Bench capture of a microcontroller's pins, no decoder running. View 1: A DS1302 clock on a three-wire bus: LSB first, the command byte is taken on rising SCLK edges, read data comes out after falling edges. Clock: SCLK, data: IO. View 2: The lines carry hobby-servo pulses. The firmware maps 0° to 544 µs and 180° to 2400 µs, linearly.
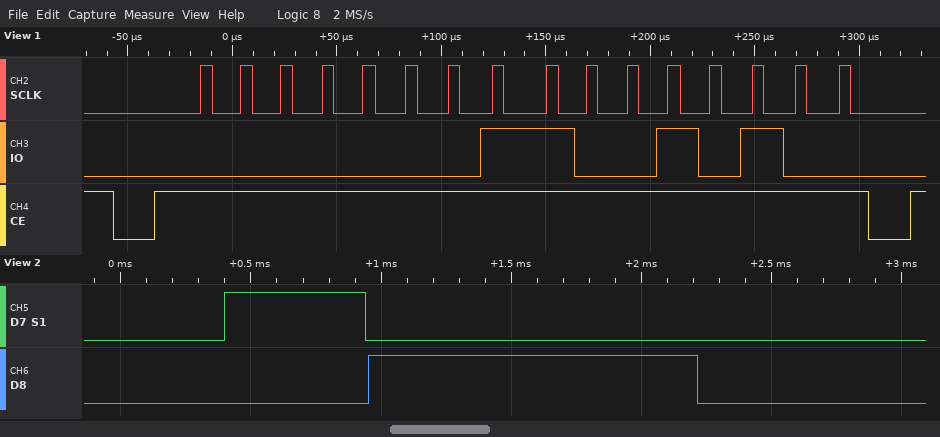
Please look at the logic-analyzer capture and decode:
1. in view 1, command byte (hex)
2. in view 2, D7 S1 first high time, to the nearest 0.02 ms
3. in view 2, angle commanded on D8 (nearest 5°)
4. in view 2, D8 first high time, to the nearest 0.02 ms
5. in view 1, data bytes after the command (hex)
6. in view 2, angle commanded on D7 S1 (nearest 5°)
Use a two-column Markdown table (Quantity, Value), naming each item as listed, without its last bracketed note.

| Quantity | Value |
|---|---|
| in view 1, command byte | 0x80 |
| in view 2, D7 S1 first high time, to the nearest 0.02 ms | 0.54 ms |
| in view 2, angle commanded on D8 | 70° |
| in view 2, D8 first high time, to the nearest 0.02 ms | 1.26 ms |
| in view 1, data bytes after the command | 29 |
| in view 2, angle commanded on D7 S1 | 0° |
